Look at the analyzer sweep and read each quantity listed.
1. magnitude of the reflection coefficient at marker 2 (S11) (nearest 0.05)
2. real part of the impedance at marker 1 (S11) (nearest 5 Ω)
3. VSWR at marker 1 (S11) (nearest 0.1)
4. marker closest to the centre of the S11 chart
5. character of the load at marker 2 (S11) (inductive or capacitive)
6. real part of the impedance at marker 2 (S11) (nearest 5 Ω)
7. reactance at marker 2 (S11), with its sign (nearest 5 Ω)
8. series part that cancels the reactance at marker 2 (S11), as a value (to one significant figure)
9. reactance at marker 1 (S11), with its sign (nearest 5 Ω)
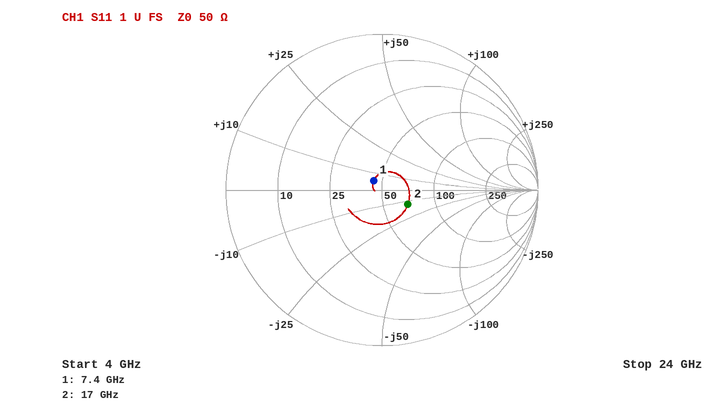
0.20
45 Ω
1.2
marker 1
capacitive
70 Ω
-15 Ω
100 pH
+5 Ω
